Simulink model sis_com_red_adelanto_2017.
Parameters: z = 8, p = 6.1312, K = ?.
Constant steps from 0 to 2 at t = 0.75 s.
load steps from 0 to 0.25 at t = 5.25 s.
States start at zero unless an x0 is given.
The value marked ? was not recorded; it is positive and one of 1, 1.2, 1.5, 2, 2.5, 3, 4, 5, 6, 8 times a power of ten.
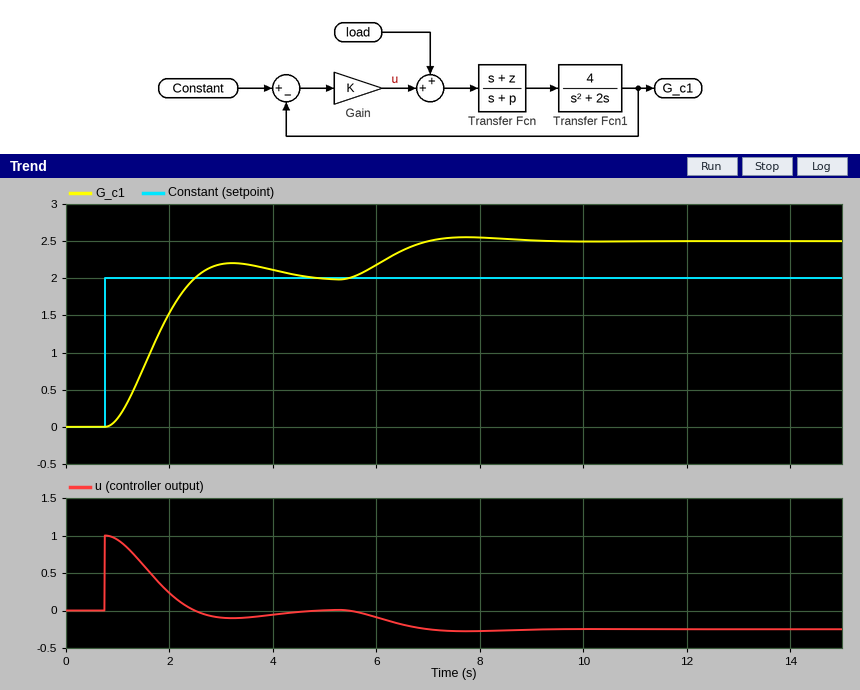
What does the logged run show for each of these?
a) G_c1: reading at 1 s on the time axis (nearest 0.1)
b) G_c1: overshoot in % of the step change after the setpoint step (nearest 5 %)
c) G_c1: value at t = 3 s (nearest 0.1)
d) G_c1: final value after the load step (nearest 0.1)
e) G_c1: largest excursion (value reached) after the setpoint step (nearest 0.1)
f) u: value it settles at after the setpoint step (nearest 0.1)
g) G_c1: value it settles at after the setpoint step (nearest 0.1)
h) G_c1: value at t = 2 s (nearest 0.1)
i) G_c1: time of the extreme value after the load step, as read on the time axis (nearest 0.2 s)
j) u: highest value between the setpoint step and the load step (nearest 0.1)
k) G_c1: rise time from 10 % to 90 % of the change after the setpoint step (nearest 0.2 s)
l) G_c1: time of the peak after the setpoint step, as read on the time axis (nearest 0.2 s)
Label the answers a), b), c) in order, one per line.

a) 0.1
b) 10 %
c) 2.2
d) 2.5
e) 2.2
f) 0.0
g) 2.0
h) 1.5
i) 7.8 s
j) 1.0
k) 1.2 s
l) 3.2 s
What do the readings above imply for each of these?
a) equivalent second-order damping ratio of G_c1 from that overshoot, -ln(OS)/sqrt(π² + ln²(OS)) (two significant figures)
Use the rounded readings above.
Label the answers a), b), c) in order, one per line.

a) 0.59
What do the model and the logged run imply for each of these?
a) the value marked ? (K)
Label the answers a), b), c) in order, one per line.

a) 0.5
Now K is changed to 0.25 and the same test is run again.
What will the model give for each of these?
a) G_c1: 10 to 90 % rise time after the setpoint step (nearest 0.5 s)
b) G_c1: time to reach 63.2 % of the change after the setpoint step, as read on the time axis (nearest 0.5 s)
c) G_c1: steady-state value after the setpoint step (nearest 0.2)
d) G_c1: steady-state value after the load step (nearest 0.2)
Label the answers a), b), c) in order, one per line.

a) 2.5 s
b) 2.5 s
c) 2.0
d) 3.0
